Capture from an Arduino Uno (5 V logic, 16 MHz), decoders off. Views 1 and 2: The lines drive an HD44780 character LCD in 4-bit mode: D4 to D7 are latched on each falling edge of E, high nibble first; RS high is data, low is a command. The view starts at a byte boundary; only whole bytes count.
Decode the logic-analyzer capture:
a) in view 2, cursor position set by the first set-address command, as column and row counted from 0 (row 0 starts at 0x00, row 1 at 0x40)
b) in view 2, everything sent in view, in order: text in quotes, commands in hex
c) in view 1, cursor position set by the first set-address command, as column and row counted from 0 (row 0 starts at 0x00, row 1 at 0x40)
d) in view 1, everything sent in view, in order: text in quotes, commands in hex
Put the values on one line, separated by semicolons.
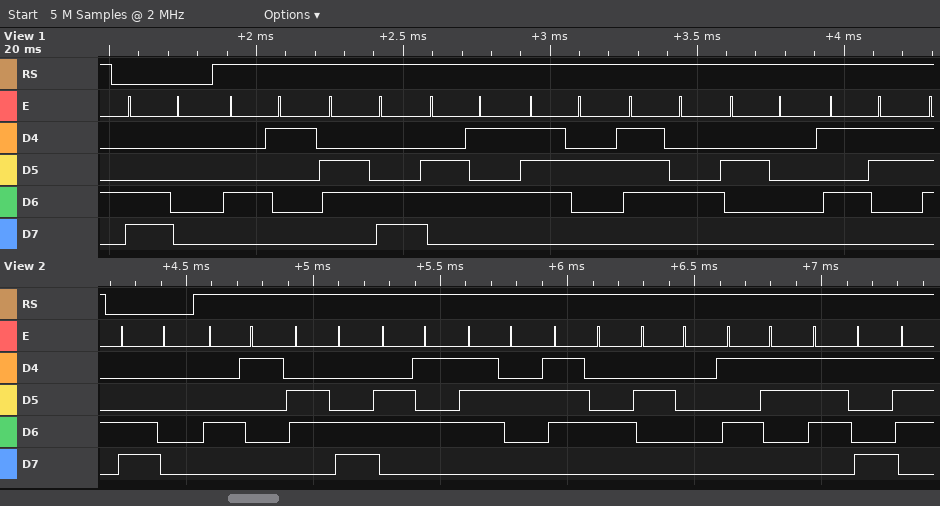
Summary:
column 0, row 1; 0xC0 "Alert Sy"; column 0, row 1; 0xC0 "Alert S"
